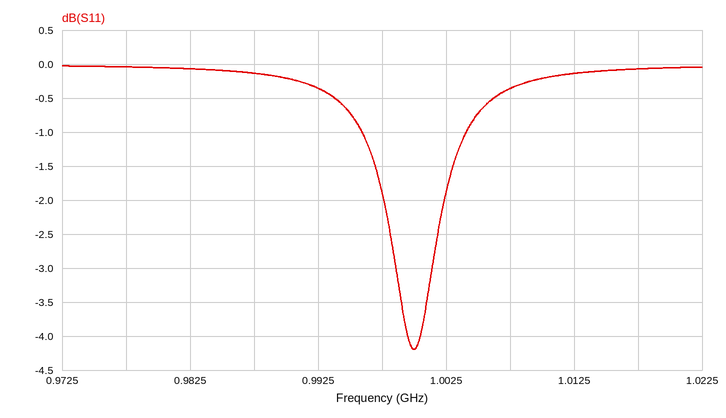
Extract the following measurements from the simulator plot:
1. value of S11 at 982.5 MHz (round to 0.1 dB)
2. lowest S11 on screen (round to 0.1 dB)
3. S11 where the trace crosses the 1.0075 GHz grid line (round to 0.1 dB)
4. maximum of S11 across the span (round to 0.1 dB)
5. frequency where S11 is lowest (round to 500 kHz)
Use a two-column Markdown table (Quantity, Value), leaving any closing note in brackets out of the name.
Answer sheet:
| Quantity | Value |
|---|---|
| value of S11 at 982.5 MHz | -0.1 dB |
| lowest S11 on screen | -4.2 dB |
| S11 where the trace crosses the 1.0075 GHz grid line | -0.4 dB |
| maximum of S11 across the span | 0.0 dB |
| frequency where S11 is lowest | 1.0000 GHz |
